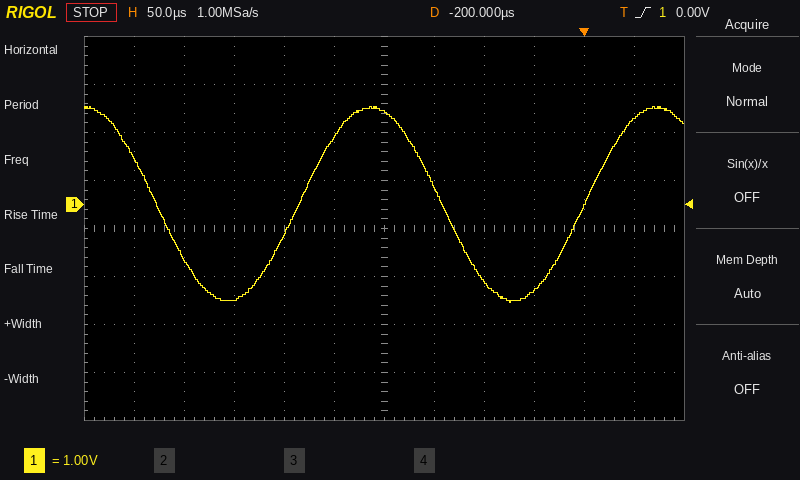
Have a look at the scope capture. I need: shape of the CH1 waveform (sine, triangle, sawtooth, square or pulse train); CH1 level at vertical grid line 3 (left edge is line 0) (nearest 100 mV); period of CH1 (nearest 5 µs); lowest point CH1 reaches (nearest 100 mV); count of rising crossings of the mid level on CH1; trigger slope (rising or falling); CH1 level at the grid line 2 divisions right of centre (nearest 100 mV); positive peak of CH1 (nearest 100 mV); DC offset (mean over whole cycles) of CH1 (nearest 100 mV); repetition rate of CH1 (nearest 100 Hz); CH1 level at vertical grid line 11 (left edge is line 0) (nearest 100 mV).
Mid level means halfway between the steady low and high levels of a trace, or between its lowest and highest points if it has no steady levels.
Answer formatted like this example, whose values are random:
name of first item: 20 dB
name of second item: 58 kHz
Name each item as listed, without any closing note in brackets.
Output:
shape of the CH1 waveform: sine
CH1 level at vertical grid line 3 (left edge is line 0): -2.0 V
period of CH1: 285 µs
lowest point CH1 reaches: -2.0 V
count of rising crossings of the mid level on CH1: 2
trigger slope: rising
CH1 level at the grid line 2 divisions right of centre: -1.6 V
positive peak of CH1: 2.0 V
DC offset (mean over whole cycles) of CH1: 0.0 V
repetition rate of CH1: 3.5 kHz
CH1 level at vertical grid line 11 (left edge is line 0): 1.8 V
